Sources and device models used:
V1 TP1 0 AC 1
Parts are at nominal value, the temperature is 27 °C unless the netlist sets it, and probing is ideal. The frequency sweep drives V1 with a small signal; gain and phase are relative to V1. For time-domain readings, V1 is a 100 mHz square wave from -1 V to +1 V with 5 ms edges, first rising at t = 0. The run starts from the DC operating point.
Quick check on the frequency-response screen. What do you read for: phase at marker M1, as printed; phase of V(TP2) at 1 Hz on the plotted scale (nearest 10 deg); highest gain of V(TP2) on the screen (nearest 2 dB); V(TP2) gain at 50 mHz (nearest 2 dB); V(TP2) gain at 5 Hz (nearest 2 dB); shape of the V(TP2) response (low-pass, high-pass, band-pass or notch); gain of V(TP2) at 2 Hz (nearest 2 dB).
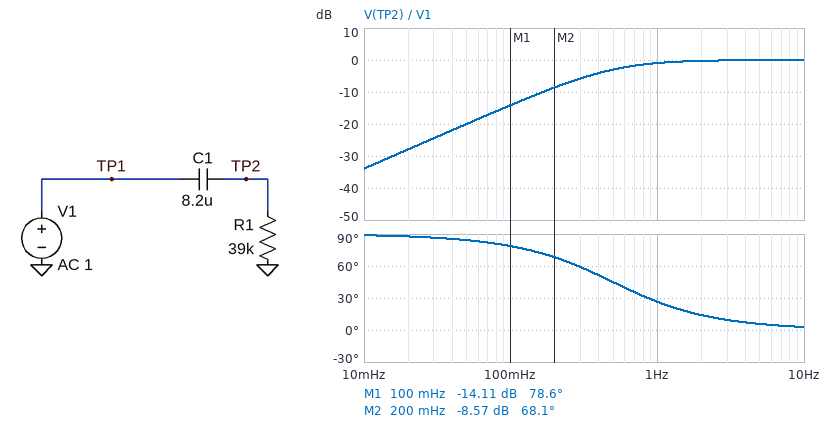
78.6 deg
30 deg
0 dB
-20 dB
0 dB
high-pass
0 dB
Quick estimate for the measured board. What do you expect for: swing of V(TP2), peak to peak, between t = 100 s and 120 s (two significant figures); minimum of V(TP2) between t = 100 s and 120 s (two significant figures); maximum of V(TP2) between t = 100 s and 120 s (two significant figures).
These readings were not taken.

4.0 V
-2.0 V
2.0 V
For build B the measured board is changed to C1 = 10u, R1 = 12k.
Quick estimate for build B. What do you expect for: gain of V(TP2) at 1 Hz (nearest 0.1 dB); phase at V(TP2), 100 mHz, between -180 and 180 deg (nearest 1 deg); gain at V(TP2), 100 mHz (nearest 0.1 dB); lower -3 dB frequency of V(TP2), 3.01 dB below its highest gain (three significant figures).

-4.4 dB
86 deg
-22.5 dB
1.33 Hz
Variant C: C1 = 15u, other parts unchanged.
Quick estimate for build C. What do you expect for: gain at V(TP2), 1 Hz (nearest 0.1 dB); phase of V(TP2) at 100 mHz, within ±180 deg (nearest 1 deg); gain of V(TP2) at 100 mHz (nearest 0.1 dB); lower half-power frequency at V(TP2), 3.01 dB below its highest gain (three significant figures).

-0.3 dB
70 deg
-9.2 dB
272 mHz
